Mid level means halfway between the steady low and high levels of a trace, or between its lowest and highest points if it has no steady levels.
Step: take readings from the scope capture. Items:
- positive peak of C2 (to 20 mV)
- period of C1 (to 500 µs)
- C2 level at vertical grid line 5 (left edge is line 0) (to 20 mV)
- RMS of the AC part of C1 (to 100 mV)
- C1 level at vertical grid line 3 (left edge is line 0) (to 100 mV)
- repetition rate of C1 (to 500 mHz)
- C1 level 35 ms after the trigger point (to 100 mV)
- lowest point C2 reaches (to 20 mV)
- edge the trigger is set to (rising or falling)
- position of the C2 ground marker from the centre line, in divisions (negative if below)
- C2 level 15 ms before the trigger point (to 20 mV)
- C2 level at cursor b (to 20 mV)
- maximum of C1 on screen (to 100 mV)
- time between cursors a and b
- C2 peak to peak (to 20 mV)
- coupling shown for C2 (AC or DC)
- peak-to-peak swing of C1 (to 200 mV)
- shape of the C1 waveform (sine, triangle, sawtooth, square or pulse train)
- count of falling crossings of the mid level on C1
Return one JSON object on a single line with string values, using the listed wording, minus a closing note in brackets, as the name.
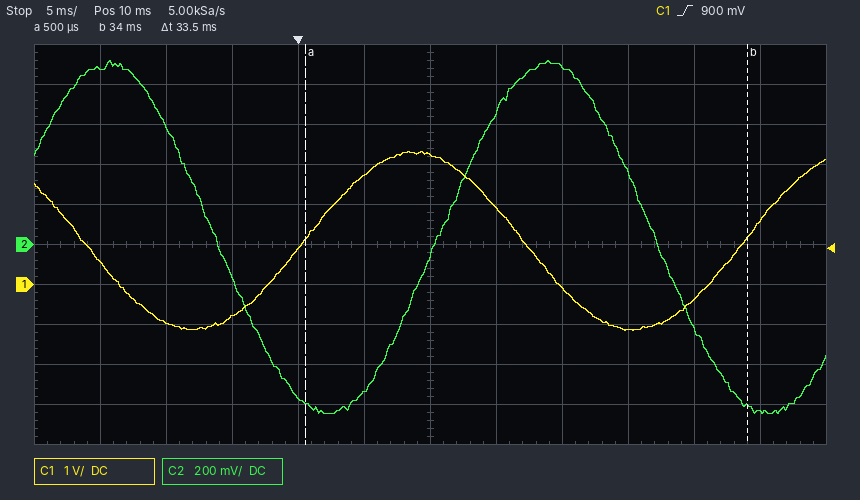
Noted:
{"positive peak of C2": "920 mV", "period of C1": "33.5 ms", "C2 level at vertical grid line 5 (left edge is line 0)": "-740 mV", "RMS of the AC part of C1": "1.6 V", "C1 level at vertical grid line 3 (left edge is line 0)": "-800 mV", "repetition rate of C1": "30.0 Hz", "C1 level 35 ms after the trigger point": "1.6 V", "lowest point C2 reaches": "-840 mV", "edge the trigger is set to": "rising", "position of the C2 ground marker from the centre line, in divisions": "0.0 div", "C2 level 15 ms before the trigger point": "880 mV", "C2 level at cursor b": "-800 mV", "maximum of C1 on screen": "3.3 V", "time between cursors a and b": "33.5 ms", "C2 peak to peak": "1.76 V", "coupling shown for C2": "DC", "peak-to-peak swing of C1": "4.4 V", "shape of the C1 waveform": "sine", "count of falling crossings of the mid level on C1": "2"}
